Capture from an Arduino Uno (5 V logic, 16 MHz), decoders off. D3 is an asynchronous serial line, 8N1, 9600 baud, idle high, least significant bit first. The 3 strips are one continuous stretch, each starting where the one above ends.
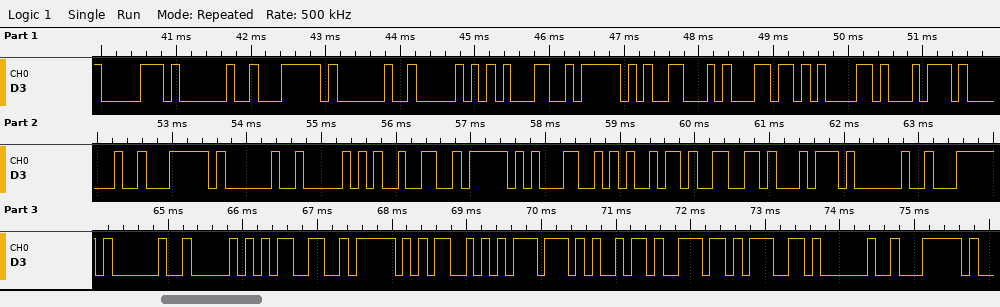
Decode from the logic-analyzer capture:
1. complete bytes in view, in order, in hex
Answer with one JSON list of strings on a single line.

["0x70 0x20 0x7C 0x20 0x50 0x31 0x5F 0x46 0x6C 0x61 0x74 0x20 0x7C 0x20 0x50 0x32 0x5F 0x4C 0x69 0x66 0x74 0x20 0x7C 0x20 0x50 0x33 0x5F 0x53 0x77 0x69 0x6E 0x67 0x20 0x7C"]
